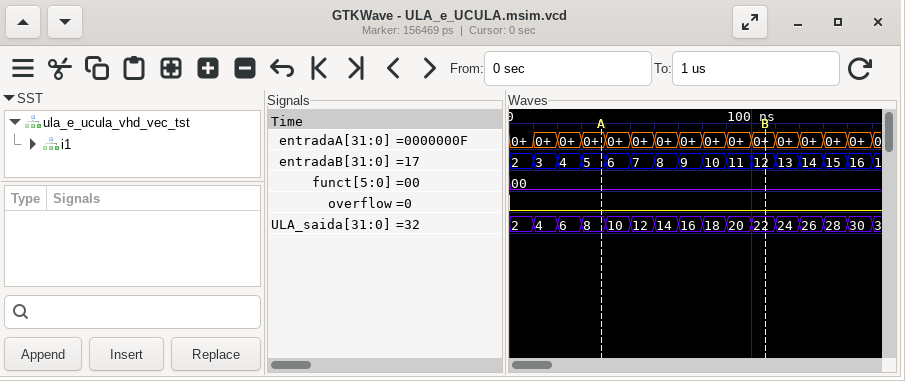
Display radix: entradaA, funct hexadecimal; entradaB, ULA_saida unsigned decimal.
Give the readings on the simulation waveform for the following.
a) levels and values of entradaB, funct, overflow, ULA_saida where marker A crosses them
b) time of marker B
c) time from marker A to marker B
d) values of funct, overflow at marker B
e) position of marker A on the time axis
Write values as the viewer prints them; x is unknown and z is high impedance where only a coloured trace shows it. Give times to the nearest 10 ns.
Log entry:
entradaB=5, funct=00, overflow=0, ULA_saida=8
110 ns
70 ns
funct=00, overflow=0
40 ns
